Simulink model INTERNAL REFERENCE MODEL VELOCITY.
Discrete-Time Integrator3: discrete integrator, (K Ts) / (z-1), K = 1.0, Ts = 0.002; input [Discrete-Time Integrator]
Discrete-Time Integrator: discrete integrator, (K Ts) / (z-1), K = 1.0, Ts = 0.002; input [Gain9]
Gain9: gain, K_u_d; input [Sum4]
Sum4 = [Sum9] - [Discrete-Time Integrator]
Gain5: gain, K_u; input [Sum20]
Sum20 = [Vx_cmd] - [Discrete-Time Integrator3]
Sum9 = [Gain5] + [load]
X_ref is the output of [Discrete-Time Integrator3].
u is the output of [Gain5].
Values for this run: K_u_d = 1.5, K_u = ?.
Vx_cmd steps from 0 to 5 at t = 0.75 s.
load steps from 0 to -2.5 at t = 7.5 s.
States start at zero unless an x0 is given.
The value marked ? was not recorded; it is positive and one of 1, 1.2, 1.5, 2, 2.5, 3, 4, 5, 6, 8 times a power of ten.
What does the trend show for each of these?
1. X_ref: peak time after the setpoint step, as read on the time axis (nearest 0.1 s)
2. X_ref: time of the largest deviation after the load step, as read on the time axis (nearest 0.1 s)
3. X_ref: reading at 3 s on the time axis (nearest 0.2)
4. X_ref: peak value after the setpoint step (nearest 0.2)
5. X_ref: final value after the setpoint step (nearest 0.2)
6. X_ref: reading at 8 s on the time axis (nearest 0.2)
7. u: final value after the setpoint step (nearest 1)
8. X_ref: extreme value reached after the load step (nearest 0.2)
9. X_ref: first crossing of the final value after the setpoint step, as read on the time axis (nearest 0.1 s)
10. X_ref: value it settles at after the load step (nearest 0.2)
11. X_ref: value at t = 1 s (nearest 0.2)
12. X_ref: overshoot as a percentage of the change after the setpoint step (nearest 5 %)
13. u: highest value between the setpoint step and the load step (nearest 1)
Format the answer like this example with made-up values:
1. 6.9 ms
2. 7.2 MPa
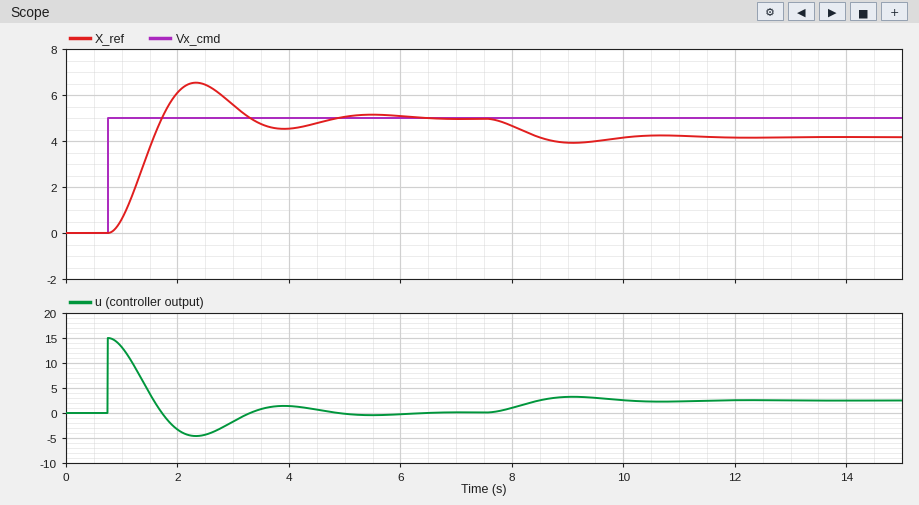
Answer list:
1. 2.3 s
2. 9.1 s
3. 5.6
4. 6.6
5. 5.0
6. 4.6
7. 0
8. 4.0
9. 1.7 s
10. 4.2
11. 0.6
12. 30 %
13. 15
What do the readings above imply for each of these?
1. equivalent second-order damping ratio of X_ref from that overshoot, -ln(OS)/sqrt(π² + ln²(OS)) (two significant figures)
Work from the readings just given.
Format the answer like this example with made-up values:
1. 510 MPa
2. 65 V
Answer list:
1. 0.36
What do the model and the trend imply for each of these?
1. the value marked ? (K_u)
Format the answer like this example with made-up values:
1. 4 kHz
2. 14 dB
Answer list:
1. 3
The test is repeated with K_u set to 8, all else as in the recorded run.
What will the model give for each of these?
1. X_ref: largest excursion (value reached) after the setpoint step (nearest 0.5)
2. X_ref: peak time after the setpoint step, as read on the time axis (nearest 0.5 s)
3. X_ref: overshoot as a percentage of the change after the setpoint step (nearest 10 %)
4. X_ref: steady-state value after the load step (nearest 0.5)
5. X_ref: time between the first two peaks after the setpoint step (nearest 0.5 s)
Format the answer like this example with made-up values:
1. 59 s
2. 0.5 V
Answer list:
1. 7.5
2. 1.5 s
3. 50 %
4. 4.5
5. 2.0 s
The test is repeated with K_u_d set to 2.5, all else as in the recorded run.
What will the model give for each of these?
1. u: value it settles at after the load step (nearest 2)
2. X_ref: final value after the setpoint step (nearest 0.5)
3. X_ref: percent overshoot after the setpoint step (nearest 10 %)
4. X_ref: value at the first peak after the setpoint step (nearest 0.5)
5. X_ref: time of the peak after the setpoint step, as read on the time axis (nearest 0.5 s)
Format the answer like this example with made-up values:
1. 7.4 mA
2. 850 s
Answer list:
1. 2
2. 5.0
3. 20 %
4. 6.0
5. 2.0 s
